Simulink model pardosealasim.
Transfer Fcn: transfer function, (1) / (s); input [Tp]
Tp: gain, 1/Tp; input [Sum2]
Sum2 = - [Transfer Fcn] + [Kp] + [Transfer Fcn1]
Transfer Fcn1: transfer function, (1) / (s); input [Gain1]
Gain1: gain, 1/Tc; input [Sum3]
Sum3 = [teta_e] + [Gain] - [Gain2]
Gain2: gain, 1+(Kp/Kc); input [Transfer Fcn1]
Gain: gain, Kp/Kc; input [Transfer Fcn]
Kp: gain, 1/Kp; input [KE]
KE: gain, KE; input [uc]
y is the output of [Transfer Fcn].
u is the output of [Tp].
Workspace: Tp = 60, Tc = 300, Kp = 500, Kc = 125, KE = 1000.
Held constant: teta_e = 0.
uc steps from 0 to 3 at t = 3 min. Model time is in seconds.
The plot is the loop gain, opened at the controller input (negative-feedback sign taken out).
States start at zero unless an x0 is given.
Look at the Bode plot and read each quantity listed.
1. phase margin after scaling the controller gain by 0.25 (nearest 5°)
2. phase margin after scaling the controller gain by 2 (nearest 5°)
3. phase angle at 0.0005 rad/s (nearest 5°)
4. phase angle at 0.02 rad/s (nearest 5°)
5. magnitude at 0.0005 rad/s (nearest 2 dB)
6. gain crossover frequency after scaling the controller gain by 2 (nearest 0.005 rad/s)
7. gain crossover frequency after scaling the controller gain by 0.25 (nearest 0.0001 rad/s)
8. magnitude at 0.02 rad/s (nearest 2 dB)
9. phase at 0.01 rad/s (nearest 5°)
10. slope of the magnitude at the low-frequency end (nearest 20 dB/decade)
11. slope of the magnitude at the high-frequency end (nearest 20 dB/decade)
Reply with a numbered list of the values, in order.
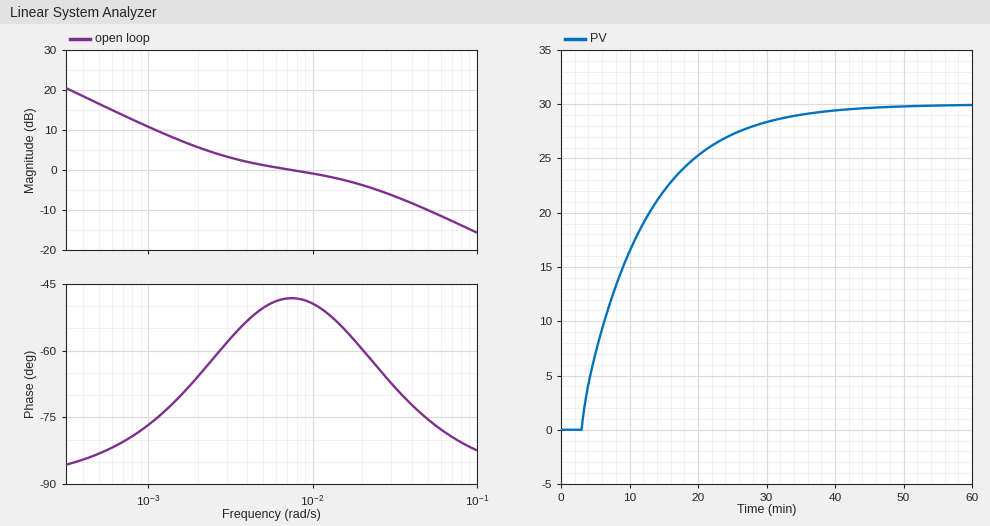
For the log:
1. 100°
2. 115°
3. -85°
4. -60°
5. 16 dB
6. 0.030 rad/s
7. 0.0009 rad/s
8. -4 dB
9. -50°
10. -20 dB/decade
11. -20 dB/decade
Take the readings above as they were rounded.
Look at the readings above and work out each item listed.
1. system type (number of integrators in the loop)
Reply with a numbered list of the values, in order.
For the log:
1. 1
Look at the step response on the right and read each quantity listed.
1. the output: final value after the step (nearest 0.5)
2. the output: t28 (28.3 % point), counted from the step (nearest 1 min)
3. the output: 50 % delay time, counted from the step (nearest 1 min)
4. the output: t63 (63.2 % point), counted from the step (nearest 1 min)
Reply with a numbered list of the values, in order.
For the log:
1. 30.0
2. 3 min
3. 6 min
4. 9 min
